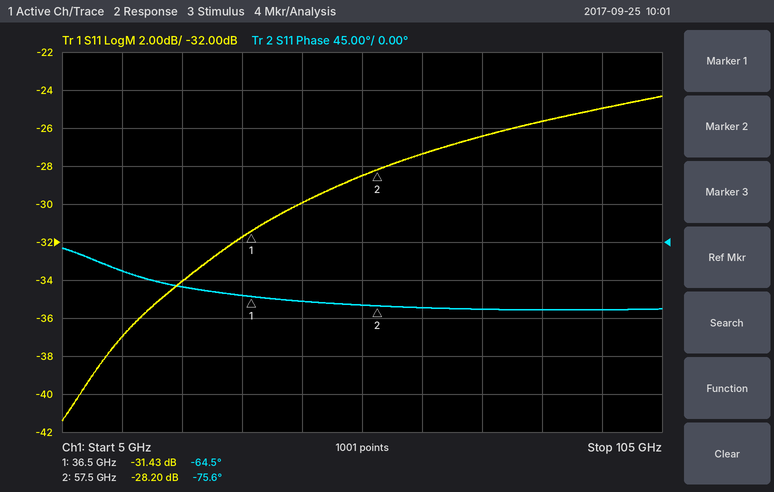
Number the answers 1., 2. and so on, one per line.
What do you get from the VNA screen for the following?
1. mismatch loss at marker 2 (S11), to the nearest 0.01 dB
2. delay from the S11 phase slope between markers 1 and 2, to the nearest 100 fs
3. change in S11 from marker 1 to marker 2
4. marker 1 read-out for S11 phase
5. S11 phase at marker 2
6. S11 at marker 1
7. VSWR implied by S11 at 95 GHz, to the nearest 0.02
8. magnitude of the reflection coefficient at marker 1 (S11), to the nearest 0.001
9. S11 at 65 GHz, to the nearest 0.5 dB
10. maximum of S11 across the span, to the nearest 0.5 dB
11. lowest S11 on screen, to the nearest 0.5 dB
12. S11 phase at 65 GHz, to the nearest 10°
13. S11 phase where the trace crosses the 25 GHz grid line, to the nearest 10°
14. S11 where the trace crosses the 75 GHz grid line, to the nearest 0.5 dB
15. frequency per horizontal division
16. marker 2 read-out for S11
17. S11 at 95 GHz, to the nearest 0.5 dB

1. 0.01 dB
2. 1.5 ps
3. 3.23 dB
4. -64.5°
5. -75.6°
6. -31.43 dB
7. 1.12
8. 0.027
9. -27.5 dB
10. -24.5 dB
11. -41.5 dB
12. -80°
13. -50°
14. -26.5 dB
15. 10 GHz
16. -28.20 dB
17. -25.0 dB
